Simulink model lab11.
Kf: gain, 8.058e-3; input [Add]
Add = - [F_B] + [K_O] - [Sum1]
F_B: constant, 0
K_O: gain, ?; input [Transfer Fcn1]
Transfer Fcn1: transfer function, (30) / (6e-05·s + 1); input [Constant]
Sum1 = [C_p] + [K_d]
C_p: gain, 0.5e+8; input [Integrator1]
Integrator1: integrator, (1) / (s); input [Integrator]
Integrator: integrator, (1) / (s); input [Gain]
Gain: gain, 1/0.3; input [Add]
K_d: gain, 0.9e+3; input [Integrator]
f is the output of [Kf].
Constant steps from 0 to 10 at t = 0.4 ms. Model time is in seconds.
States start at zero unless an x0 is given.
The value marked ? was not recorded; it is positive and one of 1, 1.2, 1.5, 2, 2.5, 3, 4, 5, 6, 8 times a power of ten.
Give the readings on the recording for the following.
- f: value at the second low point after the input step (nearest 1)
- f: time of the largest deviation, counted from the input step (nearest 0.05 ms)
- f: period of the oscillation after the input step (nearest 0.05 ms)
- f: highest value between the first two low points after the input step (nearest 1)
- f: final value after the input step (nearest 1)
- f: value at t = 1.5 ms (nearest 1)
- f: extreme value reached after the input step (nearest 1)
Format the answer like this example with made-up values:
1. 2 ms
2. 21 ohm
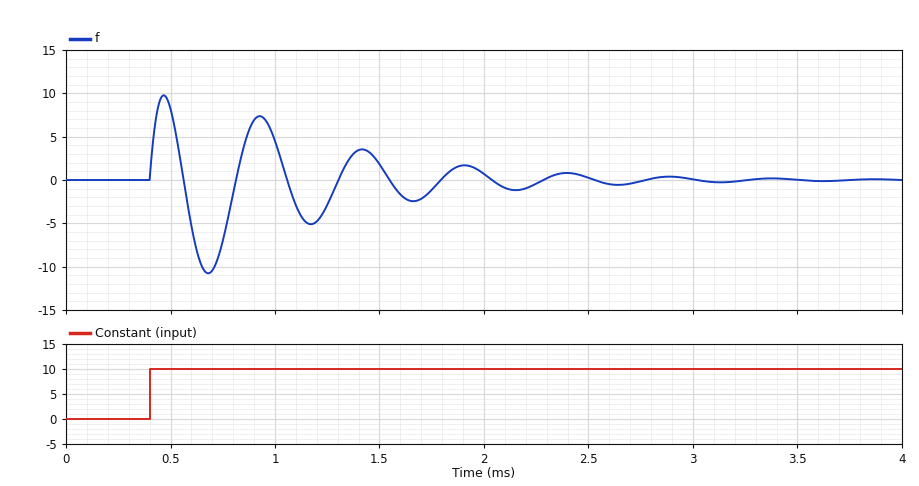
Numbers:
1. -5
2. 0.30 ms
3. 0.50 ms
4. 7
5. 0
6. 2
7. -11
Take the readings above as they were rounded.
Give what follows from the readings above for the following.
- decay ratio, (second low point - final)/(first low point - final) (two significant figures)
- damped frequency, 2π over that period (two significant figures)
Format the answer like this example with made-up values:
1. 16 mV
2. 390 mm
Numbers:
1. 0.45
2. 13 rad/ms
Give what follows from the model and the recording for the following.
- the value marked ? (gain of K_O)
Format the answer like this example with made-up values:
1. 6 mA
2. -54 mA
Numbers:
1. 8
